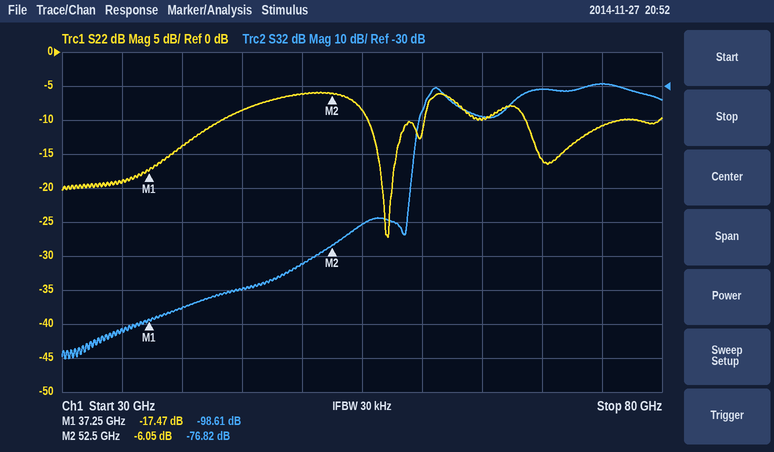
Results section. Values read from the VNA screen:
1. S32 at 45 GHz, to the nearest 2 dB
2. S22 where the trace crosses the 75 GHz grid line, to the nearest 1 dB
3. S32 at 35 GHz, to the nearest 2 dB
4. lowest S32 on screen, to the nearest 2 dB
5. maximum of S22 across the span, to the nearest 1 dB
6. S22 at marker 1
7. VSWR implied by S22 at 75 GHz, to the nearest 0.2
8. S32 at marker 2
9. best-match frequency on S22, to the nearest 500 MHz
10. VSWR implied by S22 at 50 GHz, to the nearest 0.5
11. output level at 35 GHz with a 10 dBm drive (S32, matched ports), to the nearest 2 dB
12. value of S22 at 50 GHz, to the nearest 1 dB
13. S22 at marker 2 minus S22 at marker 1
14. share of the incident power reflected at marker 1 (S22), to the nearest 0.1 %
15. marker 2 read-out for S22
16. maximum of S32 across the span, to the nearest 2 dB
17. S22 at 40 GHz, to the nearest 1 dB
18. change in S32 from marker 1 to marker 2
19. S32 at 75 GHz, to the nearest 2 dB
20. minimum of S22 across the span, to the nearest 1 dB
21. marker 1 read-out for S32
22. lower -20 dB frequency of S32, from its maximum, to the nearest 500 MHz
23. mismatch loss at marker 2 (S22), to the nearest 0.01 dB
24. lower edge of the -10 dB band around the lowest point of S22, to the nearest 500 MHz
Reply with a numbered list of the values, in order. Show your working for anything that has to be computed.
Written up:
1. -90 dB
2. -11 dB
3. -102 dB
4. -110 dB
5. -6 dB
6. -17.47 dB
7. |Γ| = 10^(-11/20) = 0.2818; VSWR = (1 + 0.2818)/(1 − 0.2818) ≈ 1.8
8. -76.82 dB
9. 57.0 GHz
10. |Γ| = 10^(-6/20) = 0.5012; VSWR = (1 + 0.5012)/(1 − 0.5012) ≈ 3.0
11. 10 dBm + (-102 dB) = -92 dBm
12. -6 dB
13. -6.05 − (-17.47) = 11.42 dB
14. 10^(-17.47/10) ≈ 1.8 %
15. -6.05 dB
16. -30 dB
17. -14 dB
18. -76.82 − (-98.61) = 21.79 dB
19. -30 dB
20. -27 dB
21. -98.61 dB
22. 59.5 GHz
23. −10 log10(1 − 10^(-6.05/10)) ≈ 1.24 dB
24. 55.5 GHz
